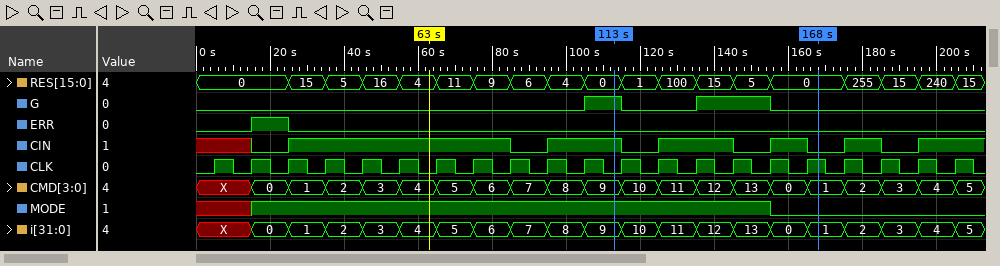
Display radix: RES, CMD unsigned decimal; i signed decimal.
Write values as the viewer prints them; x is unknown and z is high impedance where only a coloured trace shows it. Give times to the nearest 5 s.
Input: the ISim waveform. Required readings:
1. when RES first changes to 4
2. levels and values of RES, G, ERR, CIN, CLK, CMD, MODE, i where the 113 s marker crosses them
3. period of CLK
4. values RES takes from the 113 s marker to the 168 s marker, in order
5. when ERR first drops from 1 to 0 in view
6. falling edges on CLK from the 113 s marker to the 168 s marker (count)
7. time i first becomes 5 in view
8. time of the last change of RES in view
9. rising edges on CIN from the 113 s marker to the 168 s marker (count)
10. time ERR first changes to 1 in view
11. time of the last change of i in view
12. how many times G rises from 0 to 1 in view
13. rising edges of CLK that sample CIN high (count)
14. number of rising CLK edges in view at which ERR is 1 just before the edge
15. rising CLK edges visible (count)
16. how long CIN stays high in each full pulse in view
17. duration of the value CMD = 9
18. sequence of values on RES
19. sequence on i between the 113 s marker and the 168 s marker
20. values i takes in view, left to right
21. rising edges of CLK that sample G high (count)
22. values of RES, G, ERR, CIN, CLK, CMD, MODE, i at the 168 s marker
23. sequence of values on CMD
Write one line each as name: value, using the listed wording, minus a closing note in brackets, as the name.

when RES first changes to 4: 55 s
levels and values of RES, G, ERR, CIN, CLK, CMD, MODE, i where the 113 s marker crosses them: RES=0, G=1, ERR=0, CIN=1, CLK=0, CMD=9, MODE=1, i=9
period of CLK: 10 s
values RES takes from the 113 s marker to the 168 s marker, in order: 0, 1, 100, 15, 5, 0
when ERR first drops from 1 to 0 in view: 25 s
falling edges on CLK from the 113 s marker to the 168 s marker: 5
time i first becomes 5 in view: 65 s
time of the last change of RES in view: 205 s
rising edges on CIN from the 113 s marker to the 168 s marker: 2
time ERR first changes to 1 in view: 15 s
time of the last change of i in view: 205 s
how many times G rises from 0 to 1 in view: 2
rising edges of CLK that sample CIN high: 13
number of rising CLK edges in view at which ERR is 1 just before the edge: 1
rising CLK edges visible: 21
how long CIN stays high in each full pulse in view: 60 s, 20 s, 20 s, 10 s, 10 s
duration of the value CMD = 9: 10 s
sequence of values on RES: 0, 15, 5, 16, 4, 11, 9, 6, 4, 0, 1, 100, 15, 5, 0, 255, 15, 240, 15
sequence on i between the 113 s marker and the 168 s marker: 9, 10, 11, 12, 13, 0, 1
values i takes in view, left to right: X, 0, 1, 2, 3, 4, 5, 6, 7, 8, 9, 10, 11, 12, 13, 0, 1, 2, 3, 4, 5
rising edges of CLK that sample G high: 3
values of RES, G, ERR, CIN, CLK, CMD, MODE, i at the 168 s marker: RES=0, G=0, ERR=0, CIN=0, CLK=1, CMD=1, MODE=0, i=1
sequence of values on CMD: X, 0, 1, 2, 3, 4, 5, 6, 7, 8, 9, 10, 11, 12, 13, 0, 1, 2, 3, 4, 5
